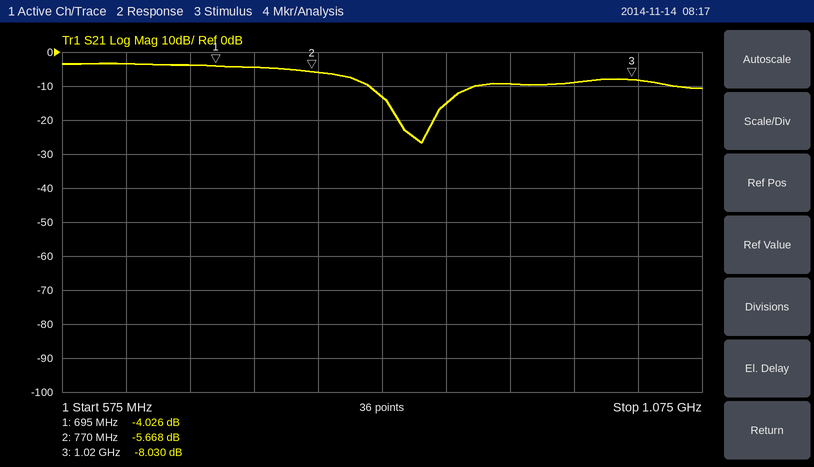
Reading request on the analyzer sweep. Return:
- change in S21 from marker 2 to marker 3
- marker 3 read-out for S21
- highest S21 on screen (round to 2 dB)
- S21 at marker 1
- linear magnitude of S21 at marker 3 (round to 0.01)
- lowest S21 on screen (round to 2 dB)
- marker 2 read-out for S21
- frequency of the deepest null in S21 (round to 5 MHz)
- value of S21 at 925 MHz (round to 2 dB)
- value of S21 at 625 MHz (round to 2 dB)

-2.362 dB
-8.030 dB
-4 dB
-4.026 dB
0.40
-26 dB
-5.668 dB
855 MHz
-10 dB
-4 dB
